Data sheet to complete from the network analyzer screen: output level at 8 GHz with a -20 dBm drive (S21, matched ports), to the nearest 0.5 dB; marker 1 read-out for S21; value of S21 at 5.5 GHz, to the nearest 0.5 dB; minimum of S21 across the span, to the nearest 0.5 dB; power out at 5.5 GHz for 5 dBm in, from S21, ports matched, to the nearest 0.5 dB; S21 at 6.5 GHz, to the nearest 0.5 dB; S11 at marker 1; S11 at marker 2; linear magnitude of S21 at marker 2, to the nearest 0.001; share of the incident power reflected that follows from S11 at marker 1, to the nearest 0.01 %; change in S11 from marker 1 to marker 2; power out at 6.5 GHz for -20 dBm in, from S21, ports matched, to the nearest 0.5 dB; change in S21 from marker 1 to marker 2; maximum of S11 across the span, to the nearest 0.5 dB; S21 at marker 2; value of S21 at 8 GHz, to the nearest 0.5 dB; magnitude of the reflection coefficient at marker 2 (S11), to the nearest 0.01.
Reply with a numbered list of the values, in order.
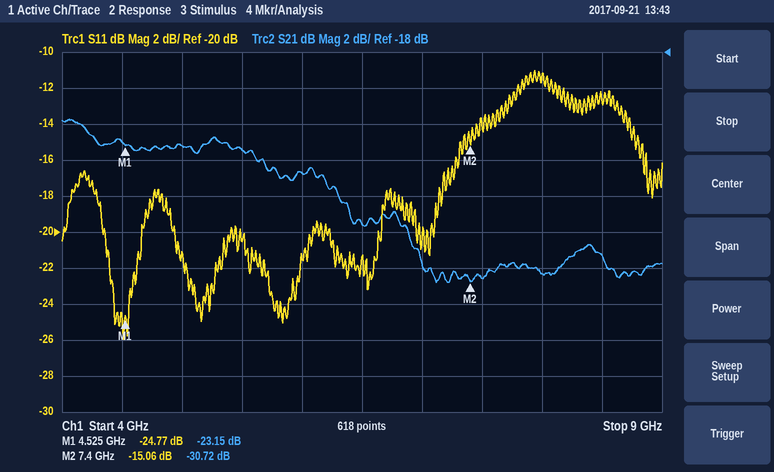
1. -50.5 dBm
2. -23.15 dB
3. -23.5 dB
4. -31.0 dB
5. -18.5 dBm
6. -27.5 dB
7. -24.77 dB
8. -15.06 dB
9. 0.029
10. 0.33 %
11. 9.71 dB
12. -47.5 dBm
13. -7.57 dB
14. -11.0 dB
15. -30.72 dB
16. -30.5 dB
17. 0.18
